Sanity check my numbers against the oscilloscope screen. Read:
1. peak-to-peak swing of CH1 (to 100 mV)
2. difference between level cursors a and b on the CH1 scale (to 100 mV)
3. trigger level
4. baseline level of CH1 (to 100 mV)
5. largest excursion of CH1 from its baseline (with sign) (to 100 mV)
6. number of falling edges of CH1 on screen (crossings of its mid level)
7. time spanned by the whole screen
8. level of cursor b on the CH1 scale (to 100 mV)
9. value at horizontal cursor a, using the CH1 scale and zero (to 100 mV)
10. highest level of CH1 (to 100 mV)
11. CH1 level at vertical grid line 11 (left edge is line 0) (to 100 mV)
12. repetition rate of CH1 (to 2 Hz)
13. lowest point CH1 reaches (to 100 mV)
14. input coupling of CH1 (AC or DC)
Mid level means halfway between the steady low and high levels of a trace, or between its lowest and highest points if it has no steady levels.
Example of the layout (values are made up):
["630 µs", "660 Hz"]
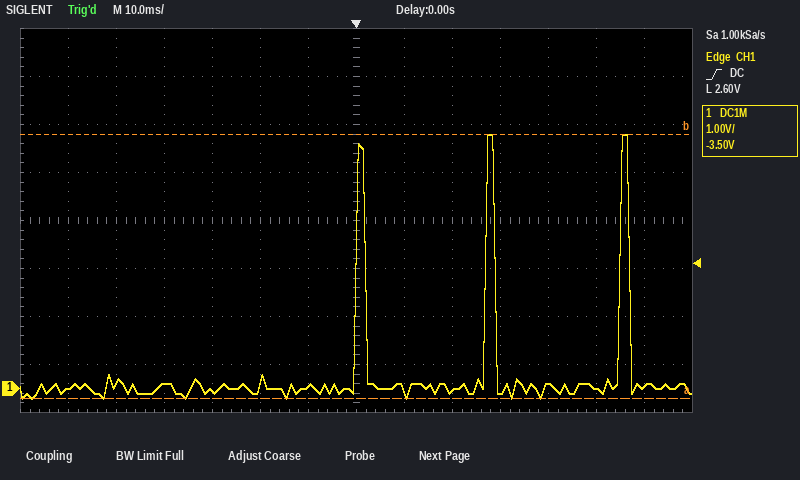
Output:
["5.5 V", "5.5 V", "2.60 V", "0.0 V", "+5.3 V", "3", "140 ms", "5.3 V", "-200 mV", "5.3 V", "100 mV", "36 Hz", "-200 mV", "DC"]
